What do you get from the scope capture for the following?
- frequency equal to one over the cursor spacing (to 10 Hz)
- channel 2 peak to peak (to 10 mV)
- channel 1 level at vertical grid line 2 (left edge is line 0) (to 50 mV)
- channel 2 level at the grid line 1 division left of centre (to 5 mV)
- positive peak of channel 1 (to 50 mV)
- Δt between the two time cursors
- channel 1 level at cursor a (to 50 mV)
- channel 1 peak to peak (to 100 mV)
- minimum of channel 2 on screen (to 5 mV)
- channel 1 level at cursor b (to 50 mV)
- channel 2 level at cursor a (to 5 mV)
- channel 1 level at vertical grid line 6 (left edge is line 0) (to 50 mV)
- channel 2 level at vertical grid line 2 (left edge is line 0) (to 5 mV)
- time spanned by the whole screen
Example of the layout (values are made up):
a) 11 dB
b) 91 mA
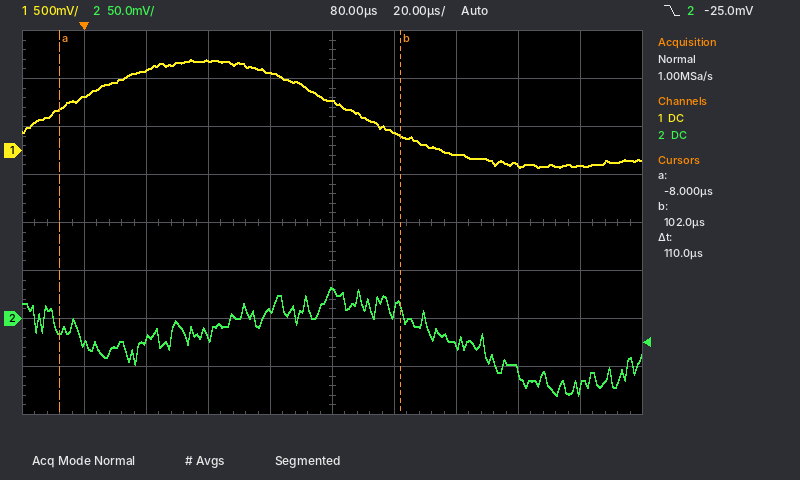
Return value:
a) 9.09 kHz
b) 110 mV
c) 850 mV
d) 10 mV
e) 950 mV
f) 110 µs
g) 450 mV
h) 1.10 V
i) -80 mV
j) 150 mV
k) -15 mV
l) 200 mV
m) -20 mV
n) 200 µs
